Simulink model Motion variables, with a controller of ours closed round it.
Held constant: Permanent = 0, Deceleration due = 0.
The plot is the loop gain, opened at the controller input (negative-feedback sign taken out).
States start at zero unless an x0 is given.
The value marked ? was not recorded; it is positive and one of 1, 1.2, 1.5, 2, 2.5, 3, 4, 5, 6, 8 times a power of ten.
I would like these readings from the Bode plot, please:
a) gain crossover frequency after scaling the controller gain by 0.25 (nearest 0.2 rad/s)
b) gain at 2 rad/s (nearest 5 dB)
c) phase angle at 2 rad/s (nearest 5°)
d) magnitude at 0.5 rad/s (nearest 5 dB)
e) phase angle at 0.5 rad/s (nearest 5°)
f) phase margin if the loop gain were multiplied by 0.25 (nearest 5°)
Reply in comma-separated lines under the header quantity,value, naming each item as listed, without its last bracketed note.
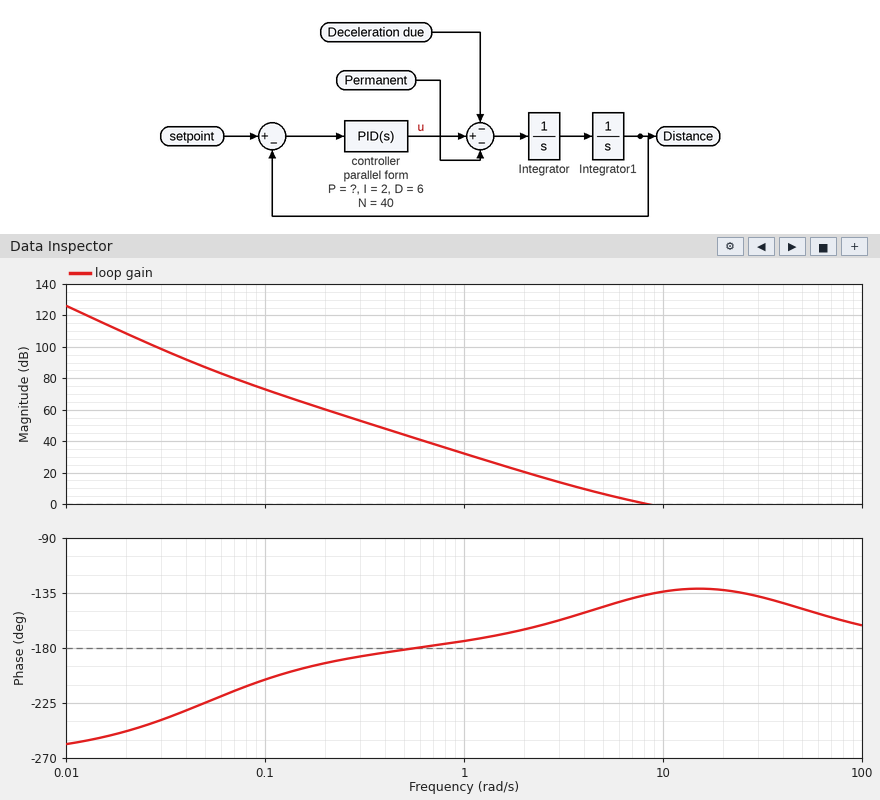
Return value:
quantity,value
gain crossover frequency after scaling the controller gain by 0.25,3.4 rad/s
gain at 2 rad/s,20 dB
phase angle at 2 rad/s,-165°
magnitude at 0.5 rad/s,45 dB
phase angle at 0.5 rad/s,-180°
phase margin if the loop gain were multiplied by 0.25,25°
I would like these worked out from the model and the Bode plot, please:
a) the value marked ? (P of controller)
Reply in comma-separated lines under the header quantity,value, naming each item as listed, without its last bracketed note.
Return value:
quantity,value
the value marked ?,40
